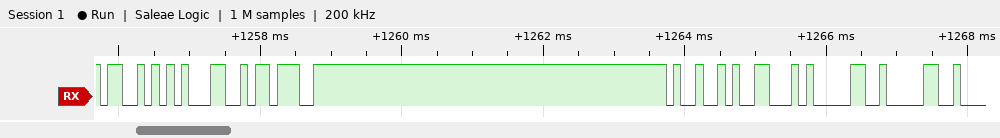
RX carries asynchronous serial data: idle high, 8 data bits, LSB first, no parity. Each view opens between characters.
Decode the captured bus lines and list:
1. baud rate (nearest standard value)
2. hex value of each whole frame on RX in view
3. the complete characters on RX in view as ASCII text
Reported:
9600 baud
53, 31, 3B, 49, 46, 30, 30
"S1;IF00"
